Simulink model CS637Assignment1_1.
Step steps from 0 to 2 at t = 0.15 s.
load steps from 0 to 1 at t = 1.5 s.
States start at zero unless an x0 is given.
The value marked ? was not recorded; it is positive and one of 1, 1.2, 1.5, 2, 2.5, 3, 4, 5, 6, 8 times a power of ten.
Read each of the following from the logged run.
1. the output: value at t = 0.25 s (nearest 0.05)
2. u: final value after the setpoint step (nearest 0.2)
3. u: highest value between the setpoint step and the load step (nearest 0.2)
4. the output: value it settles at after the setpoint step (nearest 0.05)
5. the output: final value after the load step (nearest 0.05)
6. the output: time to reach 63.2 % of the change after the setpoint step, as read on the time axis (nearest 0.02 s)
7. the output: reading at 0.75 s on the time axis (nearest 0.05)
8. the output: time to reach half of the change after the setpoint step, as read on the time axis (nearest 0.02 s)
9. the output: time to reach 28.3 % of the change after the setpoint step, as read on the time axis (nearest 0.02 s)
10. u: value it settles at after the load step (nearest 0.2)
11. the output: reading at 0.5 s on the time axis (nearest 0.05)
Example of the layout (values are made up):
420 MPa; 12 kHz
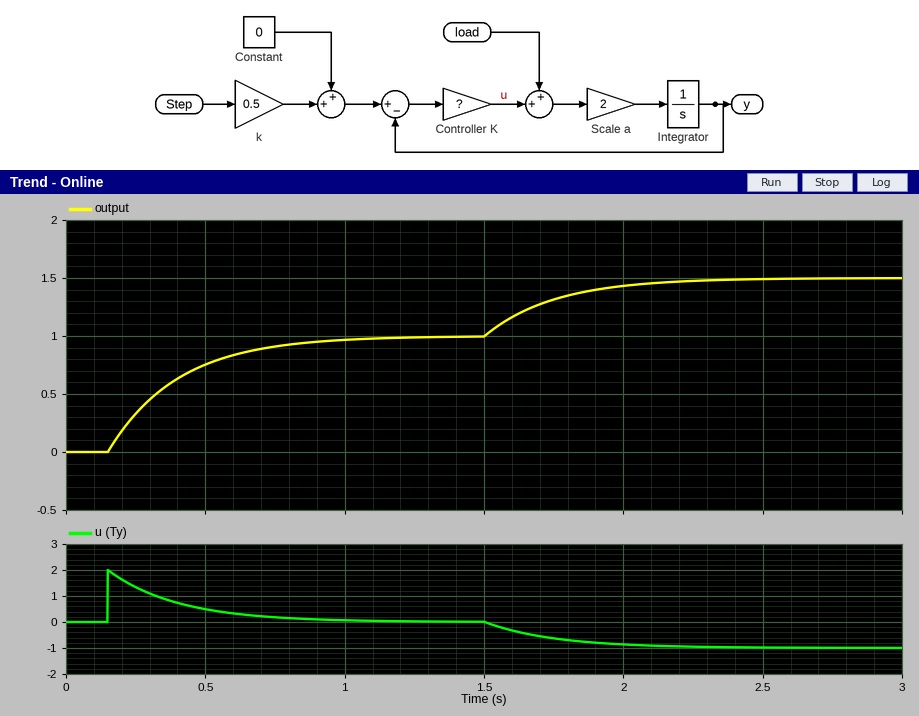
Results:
0.35; 0.0; 2.0; 1.00; 1.50; 0.40 s; 0.90; 0.32 s; 0.24 s; -1.0; 0.75
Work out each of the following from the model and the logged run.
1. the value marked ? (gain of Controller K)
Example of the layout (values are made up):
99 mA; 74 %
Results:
2
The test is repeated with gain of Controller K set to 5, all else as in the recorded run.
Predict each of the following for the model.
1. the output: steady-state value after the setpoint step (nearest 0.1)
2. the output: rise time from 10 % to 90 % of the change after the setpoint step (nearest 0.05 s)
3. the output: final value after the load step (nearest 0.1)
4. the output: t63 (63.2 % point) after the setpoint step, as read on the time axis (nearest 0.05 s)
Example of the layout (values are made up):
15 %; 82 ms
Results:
1.0; 0.20 s; 1.2; 0.25 s
